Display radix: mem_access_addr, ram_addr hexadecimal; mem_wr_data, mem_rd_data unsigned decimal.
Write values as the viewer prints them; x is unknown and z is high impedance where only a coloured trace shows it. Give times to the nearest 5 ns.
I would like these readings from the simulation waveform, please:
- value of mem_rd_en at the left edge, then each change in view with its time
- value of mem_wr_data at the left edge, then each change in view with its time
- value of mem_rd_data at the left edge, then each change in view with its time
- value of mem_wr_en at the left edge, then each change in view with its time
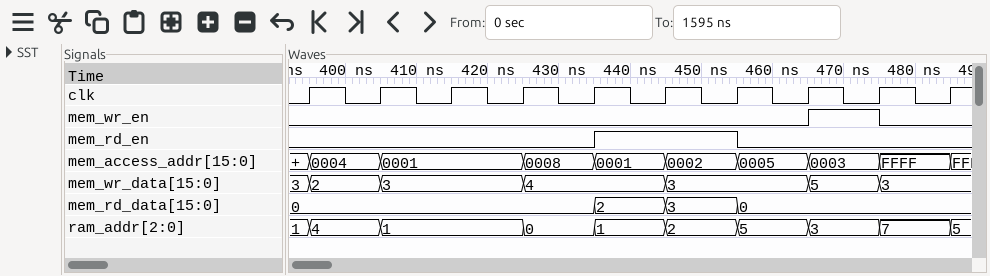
0, 1 at 435 ns, 0 at 455 ns
3, 2 at 395 ns, 3 at 405 ns, 4 at 425 ns, 3 at 445 ns, 5 at 465 ns, 3 at 475 ns
0, 2 at 435 ns, 3 at 445 ns, 0 at 455 ns
0, 1 at 465 ns, 0 at 475 ns
